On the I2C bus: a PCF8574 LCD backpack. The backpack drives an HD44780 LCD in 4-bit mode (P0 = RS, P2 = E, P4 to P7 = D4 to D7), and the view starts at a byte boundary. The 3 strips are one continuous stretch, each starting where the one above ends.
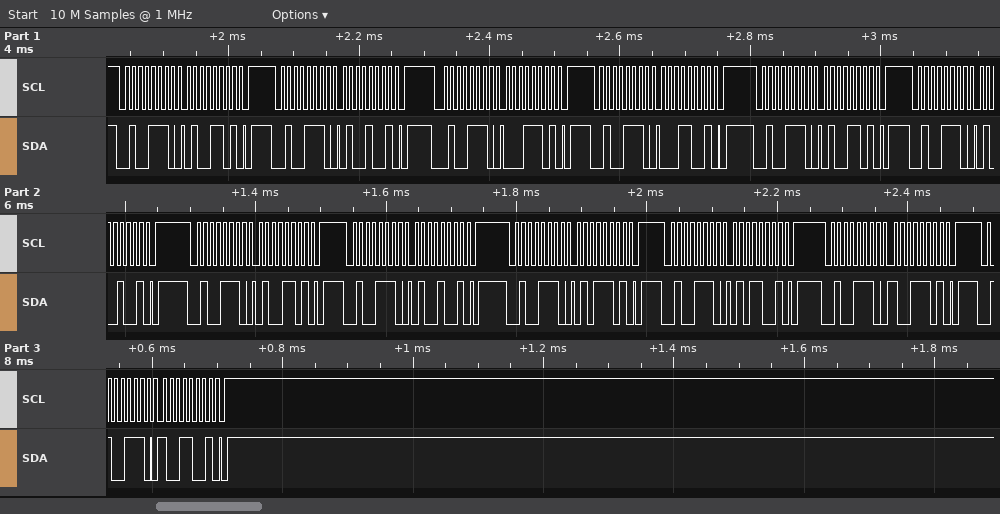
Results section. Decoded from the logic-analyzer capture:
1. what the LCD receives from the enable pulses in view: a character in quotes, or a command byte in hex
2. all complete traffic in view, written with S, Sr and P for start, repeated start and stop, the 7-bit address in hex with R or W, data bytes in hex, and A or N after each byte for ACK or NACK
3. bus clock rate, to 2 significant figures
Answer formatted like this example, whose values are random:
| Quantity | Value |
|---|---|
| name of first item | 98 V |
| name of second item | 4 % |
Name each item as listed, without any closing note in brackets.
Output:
| Quantity | Value |
|---|---|
| what the LCD receives from the enable pulses in view: a character in quotes, or a command byte in hex | 'A' 'D' 'Y' |
| all complete traffic in view, written with S, Sr and P for start, repeated start and stop, the 7-bit address in hex with R or W, data bytes in hex, and A or N after each byte for ACK or NACK | S 27W A 4D A P S 27W A 49 A P S 27W A 1D A P S 27W A 19 A P S 27W A 4D A P S 27W A 49 A P S 27W A 4D A P S 27W A 49 A P S 27W A 5D A P S 27W A 59 A P S 27W A 9D A P S 27W A 99 A P |
| bus clock rate, to 2 significant figures | 100 kHz |
